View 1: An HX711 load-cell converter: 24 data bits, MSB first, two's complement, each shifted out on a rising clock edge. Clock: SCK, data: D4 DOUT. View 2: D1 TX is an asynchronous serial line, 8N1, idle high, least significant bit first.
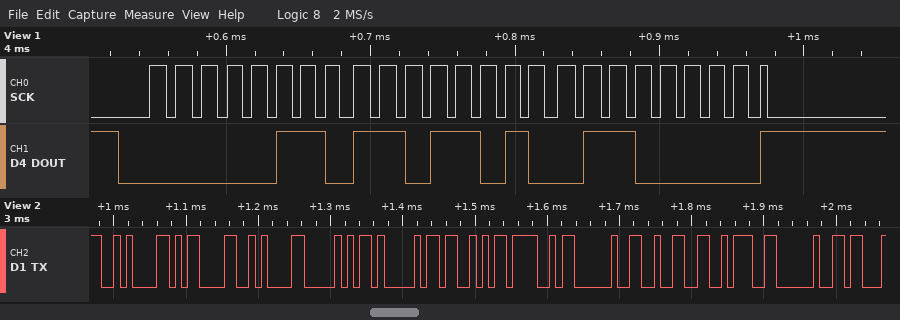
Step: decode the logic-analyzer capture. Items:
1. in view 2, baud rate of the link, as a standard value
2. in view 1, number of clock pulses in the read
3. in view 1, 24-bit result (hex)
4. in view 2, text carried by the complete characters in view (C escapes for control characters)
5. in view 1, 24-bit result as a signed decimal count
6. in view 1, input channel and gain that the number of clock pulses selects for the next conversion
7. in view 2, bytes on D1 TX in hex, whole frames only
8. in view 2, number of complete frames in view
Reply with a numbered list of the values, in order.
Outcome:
1. 115200 baud
2. 25
3. 0x06DA60
4. "\n\r\nPASO 2: "
5. 449120
6. channel A, gain 128
7. 0A 0D 0A 50 41 53 4F 20 32 3A 20
8. 11
